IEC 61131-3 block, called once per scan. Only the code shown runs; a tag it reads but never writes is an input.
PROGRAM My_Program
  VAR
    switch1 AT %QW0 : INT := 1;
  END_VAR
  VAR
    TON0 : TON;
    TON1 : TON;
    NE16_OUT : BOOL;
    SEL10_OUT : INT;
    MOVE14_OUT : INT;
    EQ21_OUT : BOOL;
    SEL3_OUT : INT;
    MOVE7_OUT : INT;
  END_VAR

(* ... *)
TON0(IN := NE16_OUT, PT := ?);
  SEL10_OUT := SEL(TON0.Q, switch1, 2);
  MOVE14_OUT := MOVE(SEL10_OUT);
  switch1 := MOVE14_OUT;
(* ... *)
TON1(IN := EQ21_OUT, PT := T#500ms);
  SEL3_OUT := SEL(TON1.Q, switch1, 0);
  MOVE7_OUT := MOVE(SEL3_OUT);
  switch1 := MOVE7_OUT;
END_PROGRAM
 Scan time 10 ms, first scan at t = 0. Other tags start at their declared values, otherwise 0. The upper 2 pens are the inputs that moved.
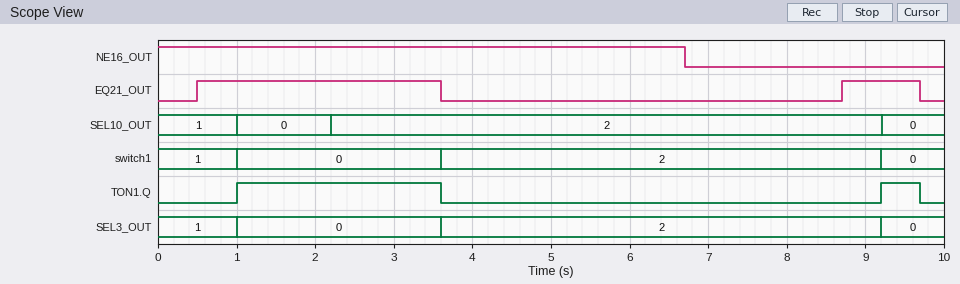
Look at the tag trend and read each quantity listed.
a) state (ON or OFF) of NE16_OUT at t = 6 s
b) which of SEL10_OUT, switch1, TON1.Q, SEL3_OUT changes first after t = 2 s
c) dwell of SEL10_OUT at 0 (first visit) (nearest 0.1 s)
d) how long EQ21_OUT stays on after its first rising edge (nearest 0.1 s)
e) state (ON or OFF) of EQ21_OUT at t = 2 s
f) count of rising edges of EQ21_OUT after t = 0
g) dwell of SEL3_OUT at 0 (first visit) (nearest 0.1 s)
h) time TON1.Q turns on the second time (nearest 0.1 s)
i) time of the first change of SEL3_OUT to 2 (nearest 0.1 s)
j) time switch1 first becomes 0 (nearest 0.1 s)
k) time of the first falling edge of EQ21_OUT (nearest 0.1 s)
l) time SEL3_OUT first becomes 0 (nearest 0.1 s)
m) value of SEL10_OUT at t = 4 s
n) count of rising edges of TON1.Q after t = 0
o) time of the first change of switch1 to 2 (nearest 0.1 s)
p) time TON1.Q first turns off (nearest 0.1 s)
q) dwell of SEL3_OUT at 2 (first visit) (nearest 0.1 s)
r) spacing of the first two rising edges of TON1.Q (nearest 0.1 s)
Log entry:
ON
SEL10_OUT
1.2 s
3.1 s
ON
2
2.6 s
9.2 s
3.6 s
1.0 s
3.6 s
1.0 s
2
2
3.6 s
3.6 s
5.6 s
8.2 s
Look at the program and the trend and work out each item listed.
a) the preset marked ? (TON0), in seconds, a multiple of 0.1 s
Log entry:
2.2 s
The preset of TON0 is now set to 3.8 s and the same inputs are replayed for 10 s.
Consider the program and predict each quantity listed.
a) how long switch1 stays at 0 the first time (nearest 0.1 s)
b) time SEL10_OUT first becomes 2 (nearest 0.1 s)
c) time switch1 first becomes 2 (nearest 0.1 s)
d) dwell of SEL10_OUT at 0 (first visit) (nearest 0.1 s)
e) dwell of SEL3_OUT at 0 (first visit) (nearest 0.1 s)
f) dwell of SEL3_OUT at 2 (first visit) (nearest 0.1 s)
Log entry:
2.8 s
3.8 s
3.8 s
2.8 s
2.8 s
5.4 s
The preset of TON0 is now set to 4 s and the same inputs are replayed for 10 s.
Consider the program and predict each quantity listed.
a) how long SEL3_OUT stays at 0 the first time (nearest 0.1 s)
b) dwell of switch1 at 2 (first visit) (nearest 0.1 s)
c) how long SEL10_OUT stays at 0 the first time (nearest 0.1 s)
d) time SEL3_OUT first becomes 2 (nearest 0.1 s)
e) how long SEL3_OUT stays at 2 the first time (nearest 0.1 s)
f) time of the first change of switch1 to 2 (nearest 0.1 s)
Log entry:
3.0 s
5.2 s
3.0 s
4.0 s
5.2 s
4.0 s
